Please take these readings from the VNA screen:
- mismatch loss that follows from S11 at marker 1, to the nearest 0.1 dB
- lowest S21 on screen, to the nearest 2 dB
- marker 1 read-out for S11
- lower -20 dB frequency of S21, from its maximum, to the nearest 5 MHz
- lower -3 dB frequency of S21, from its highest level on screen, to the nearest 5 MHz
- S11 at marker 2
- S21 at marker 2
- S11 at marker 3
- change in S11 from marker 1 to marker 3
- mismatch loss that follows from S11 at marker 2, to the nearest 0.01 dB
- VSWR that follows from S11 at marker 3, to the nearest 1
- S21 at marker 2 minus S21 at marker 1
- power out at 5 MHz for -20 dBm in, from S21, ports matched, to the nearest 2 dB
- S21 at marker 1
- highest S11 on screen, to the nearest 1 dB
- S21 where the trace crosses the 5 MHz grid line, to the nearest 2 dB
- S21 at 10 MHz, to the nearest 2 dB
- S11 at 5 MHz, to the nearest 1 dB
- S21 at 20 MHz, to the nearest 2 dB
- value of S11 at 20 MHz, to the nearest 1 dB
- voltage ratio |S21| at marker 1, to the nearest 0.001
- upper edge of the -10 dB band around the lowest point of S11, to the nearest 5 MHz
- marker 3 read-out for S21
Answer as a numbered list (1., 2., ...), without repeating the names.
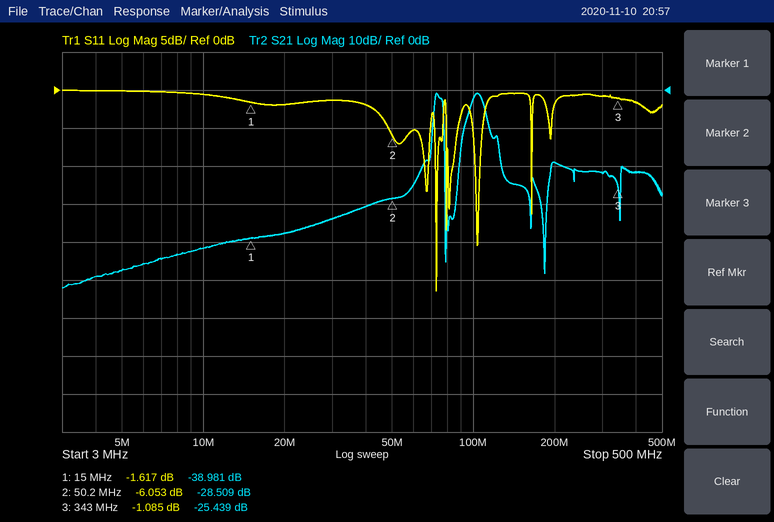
1. 5.1 dB
2. -52 dB
3. -1.617 dB
4. 65 MHz
5. 70 MHz
6. -6.053 dB
7. -28.509 dB
8. -1.085 dB
9. 0.532 dB
10. 1.24 dB
11. 16
12. 10.472 dB
13. -68 dBm
14. -38.981 dB
15. 0 dB
16. -48 dB
17. -42 dB
18. 0 dB
19. -38 dB
20. -2 dB
21. 0.011
22. 75 MHz
23. -25.439 dB
